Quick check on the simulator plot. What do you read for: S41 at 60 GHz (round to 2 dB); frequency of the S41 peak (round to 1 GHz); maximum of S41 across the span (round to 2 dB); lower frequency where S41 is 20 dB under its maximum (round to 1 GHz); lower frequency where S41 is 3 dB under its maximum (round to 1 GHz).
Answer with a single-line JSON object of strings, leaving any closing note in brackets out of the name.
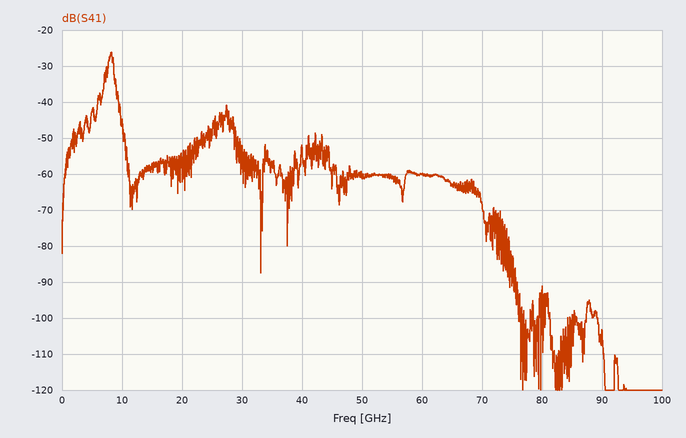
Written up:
{"S41 at 60 GHz": "-60 dB", "frequency of the S41 peak": "8 GHz", "maximum of S41 across the span": "-26 dB", "lower frequency where S41 is 20 dB under its maximum": "5 GHz", "lower frequency where S41 is 3 dB under its maximum": "8 GHz"}
